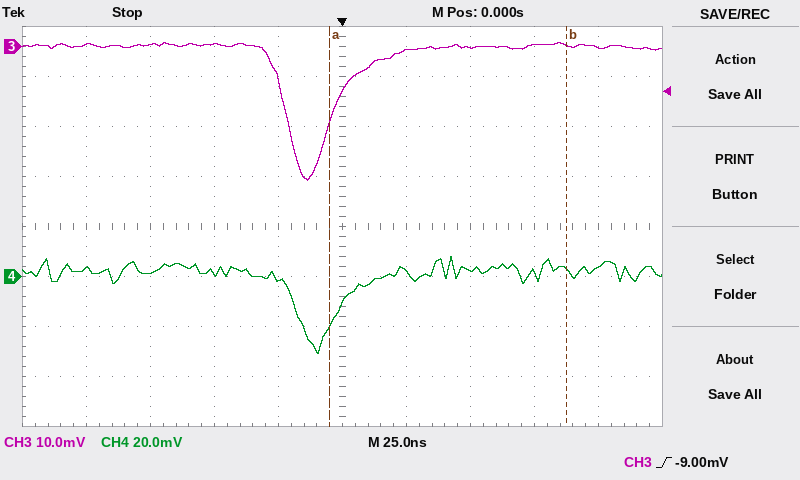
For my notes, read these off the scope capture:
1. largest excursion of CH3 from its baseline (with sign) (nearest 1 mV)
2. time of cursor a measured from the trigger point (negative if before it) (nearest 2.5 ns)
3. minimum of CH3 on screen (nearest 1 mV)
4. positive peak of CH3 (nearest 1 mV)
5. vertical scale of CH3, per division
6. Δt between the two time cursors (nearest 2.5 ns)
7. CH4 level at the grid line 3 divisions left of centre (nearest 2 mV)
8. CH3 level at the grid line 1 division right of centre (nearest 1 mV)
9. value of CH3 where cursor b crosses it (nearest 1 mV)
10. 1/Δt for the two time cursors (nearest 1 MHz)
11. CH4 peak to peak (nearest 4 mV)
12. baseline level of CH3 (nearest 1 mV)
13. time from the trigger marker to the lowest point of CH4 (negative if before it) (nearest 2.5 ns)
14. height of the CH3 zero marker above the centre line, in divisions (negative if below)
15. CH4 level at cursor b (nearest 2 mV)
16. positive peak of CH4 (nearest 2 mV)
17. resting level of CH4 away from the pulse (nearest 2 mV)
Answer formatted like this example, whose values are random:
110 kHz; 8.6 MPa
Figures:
-27 mV; -5.0 ns; -27 mV; 1 mV; 10 mV; 92.5 ns; 2 mV; -1 mV; 0 mV; 11 MHz; 40 mV; 0 mV; -10.0 ns; +3.6 div; 2 mV; 8 mV; 2 mV
